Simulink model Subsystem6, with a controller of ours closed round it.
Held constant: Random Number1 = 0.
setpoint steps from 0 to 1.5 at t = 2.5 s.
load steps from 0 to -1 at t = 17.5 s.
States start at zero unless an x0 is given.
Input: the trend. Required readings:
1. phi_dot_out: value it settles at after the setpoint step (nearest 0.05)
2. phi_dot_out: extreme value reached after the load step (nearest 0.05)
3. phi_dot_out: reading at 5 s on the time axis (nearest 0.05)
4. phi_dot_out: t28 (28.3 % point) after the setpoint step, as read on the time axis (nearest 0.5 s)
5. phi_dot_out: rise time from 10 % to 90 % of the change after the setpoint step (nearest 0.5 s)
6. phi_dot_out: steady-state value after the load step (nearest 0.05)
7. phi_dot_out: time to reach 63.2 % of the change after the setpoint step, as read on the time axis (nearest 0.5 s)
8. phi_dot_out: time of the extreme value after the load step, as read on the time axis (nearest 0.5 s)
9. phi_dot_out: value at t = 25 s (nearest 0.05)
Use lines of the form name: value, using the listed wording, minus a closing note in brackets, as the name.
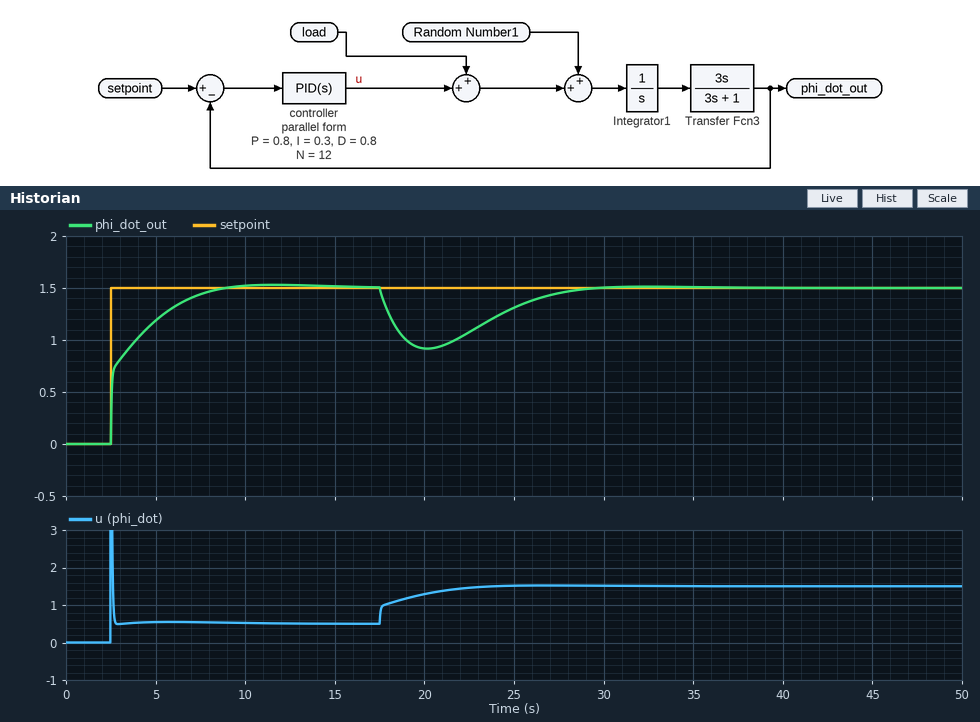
phi_dot_out: value it settles at after the setpoint step: 1.50
phi_dot_out: extreme value reached after the load step: 0.90
phi_dot_out: reading at 5 s on the time axis: 1.20
phi_dot_out: t28 (28.3 % point) after the setpoint step, as read on the time axis: 2.5 s
phi_dot_out: rise time from 10 % to 90 % of the change after the setpoint step: 4.0 s
phi_dot_out: steady-state value after the load step: 1.50
phi_dot_out: time to reach 63.2 % of the change after the setpoint step, as read on the time axis: 3.5 s
phi_dot_out: time of the extreme value after the load step, as read on the time axis: 20.0 s
phi_dot_out: value at t = 25 s: 1.30
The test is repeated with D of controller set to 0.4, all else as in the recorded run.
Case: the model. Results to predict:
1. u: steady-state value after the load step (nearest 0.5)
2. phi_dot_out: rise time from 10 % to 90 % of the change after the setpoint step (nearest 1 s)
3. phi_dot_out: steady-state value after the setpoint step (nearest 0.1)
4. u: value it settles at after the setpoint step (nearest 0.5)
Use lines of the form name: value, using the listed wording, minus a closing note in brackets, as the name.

u: steady-state value after the load step: 1.5
phi_dot_out: rise time from 10 % to 90 % of the change after the setpoint step: 3 s
phi_dot_out: steady-state value after the setpoint step: 1.5
u: value it settles at after the setpoint step: 0.5
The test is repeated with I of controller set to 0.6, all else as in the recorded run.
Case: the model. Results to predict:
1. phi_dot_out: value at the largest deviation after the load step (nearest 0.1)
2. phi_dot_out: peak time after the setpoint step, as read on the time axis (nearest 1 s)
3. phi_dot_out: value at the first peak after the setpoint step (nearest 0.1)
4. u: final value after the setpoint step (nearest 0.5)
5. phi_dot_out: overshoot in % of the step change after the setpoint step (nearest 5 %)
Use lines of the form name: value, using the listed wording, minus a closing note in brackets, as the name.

phi_dot_out: value at the largest deviation after the load step: 1.0
phi_dot_out: peak time after the setpoint step, as read on the time axis: 8 s
phi_dot_out: value at the first peak after the setpoint step: 1.6
u: final value after the setpoint step: 0.5
phi_dot_out: overshoot in % of the step change after the setpoint step: 10 %
